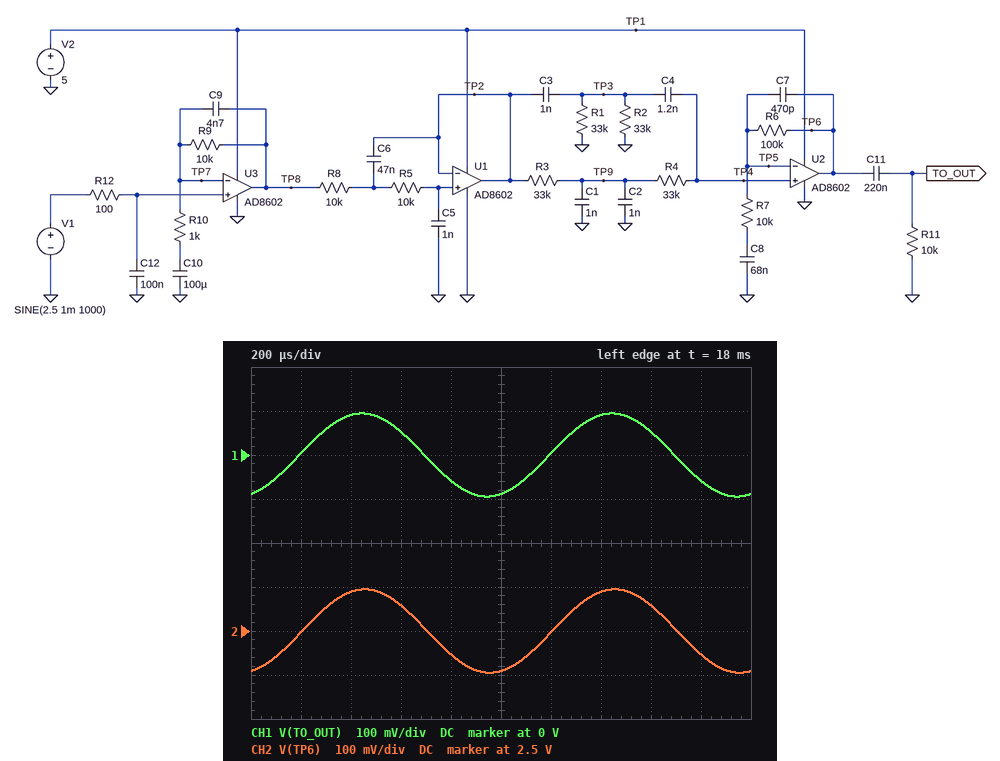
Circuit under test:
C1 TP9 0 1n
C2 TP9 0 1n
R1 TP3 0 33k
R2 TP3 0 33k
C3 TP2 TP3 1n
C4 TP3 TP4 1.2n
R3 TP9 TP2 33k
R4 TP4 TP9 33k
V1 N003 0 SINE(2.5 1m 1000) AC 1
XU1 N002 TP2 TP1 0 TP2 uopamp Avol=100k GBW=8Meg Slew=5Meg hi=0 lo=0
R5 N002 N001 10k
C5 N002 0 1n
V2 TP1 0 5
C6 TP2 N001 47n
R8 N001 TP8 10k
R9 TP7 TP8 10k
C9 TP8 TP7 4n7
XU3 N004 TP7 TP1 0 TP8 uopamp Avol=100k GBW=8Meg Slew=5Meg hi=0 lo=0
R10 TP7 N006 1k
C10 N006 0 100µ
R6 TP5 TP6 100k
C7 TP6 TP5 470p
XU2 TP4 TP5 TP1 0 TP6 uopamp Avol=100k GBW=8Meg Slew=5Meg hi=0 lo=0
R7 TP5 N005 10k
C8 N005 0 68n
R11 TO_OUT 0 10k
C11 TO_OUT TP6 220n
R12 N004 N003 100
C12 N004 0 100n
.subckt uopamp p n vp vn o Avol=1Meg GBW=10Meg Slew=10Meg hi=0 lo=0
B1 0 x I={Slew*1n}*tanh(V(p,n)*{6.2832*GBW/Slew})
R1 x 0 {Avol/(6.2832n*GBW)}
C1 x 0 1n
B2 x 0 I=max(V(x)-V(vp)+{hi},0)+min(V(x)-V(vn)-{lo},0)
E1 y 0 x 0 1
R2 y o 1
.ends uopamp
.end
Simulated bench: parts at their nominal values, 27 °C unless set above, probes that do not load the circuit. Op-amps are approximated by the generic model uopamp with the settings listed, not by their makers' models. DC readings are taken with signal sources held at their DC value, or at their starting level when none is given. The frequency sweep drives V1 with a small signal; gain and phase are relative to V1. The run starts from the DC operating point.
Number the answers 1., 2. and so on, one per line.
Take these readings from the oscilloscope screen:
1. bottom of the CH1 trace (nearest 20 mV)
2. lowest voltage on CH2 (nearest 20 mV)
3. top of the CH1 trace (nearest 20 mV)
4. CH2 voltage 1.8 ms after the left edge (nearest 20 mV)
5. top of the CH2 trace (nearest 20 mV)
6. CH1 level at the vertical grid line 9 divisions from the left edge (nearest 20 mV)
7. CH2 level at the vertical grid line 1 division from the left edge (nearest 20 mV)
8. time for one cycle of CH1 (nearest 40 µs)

1. -100 mV
2. 2.40 V
3. 100 mV
4. 2.44 V
5. 2.60 V
6. -60 mV
7. 2.50 V
8. 1.00 ms
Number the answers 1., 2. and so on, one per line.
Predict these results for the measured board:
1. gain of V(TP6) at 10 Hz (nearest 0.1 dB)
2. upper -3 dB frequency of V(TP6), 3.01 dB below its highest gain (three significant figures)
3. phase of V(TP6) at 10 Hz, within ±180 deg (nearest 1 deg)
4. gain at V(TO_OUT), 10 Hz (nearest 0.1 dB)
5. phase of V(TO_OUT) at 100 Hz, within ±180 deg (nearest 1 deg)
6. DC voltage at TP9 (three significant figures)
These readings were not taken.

1. 21.6 dB
2. 2.44 kHz
3. 30 deg
4. 4.3 dB
5. 82 deg
6. 2.50 V
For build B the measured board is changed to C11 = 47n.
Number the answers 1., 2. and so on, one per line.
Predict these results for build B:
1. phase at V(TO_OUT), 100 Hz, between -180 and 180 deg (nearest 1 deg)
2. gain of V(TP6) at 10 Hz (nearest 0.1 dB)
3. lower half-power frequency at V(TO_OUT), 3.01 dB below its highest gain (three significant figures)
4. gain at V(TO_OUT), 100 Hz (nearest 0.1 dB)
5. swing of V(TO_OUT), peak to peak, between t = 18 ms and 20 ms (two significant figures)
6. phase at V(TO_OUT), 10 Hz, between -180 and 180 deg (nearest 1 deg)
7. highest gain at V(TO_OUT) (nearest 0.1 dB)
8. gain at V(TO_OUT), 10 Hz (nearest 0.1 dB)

1. 120 deg
2. 21.6 dB
3. 358 Hz
4. 22.8 dB
5. 180 mV
6. 118 deg
7. 40.1 dB
8. -9.0 dB
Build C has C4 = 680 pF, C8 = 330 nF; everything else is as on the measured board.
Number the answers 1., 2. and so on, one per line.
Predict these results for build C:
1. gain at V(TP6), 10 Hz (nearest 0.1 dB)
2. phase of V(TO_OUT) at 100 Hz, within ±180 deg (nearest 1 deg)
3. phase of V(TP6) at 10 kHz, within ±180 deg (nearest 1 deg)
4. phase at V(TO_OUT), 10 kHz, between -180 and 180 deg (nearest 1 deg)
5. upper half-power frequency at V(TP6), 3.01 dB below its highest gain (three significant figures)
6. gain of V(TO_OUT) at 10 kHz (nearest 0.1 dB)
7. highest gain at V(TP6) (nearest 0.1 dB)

1. 28.5 dB
2. 52 deg
3. 115 deg
4. 116 deg
5. 2.47 kHz
6. -14.1 dB
7. 43.0 dB
